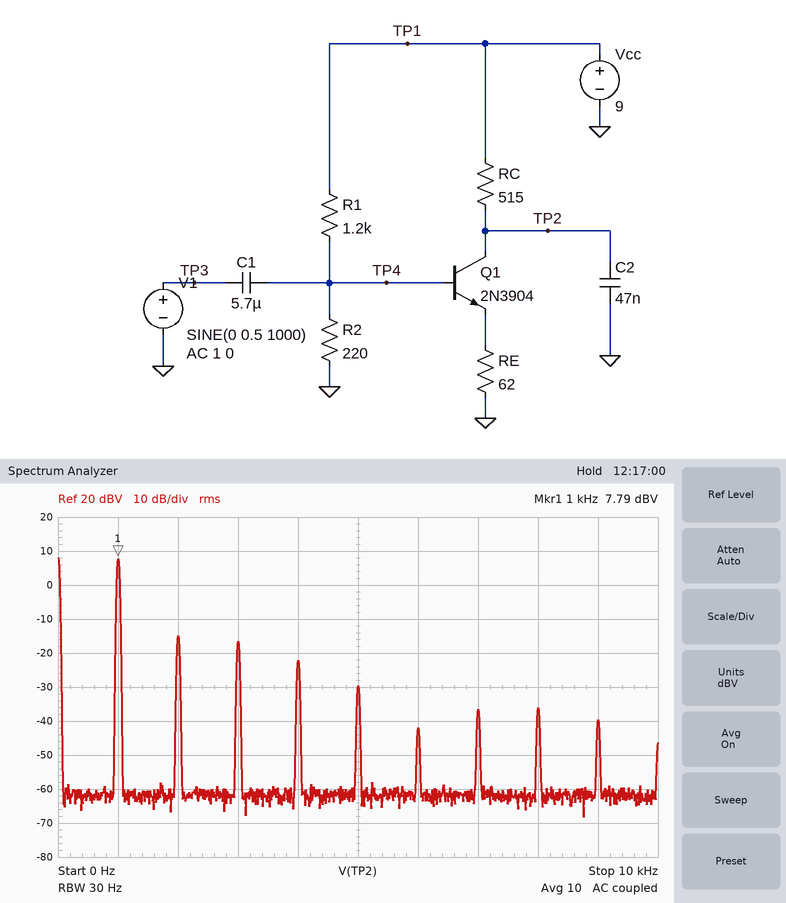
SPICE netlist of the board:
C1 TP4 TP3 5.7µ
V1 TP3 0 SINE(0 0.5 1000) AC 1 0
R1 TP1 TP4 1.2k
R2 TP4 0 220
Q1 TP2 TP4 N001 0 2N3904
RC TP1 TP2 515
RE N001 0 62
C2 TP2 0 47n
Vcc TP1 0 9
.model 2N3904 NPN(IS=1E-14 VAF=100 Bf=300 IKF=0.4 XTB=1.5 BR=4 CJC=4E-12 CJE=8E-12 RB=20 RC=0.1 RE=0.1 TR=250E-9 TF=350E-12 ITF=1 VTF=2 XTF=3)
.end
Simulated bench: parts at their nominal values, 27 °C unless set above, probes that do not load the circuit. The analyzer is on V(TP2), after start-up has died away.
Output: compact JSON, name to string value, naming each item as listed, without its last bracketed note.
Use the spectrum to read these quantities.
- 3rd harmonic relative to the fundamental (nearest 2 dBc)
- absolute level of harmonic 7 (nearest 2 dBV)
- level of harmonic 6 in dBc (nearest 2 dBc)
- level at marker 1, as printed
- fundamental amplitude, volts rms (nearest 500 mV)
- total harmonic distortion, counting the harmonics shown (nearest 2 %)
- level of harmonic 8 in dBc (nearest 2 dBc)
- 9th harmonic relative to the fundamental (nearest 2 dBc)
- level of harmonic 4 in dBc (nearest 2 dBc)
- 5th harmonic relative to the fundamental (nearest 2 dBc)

{"3rd harmonic relative to the fundamental": "-24 dBc", "absolute level of harmonic 7": "-36 dBV", "level of harmonic 6 in dBc": "-50 dBc", "level at marker 1, as printed": "7.79 dBV", "fundamental amplitude, volts rms": "2.5 V", "total harmonic distortion, counting the harmonics shown": "10 %", "level of harmonic 8 in dBc": "-44 dBc", "9th harmonic relative to the fundamental": "-48 dBc", "level of harmonic 4 in dBc": "-30 dBc", "5th harmonic relative to the fundamental": "-38 dBc"}
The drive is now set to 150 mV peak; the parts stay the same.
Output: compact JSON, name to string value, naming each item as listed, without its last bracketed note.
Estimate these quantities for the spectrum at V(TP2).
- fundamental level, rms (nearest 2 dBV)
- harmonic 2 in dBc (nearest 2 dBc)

{"fundamental level, rms": "-2 dBV", "harmonic 2 in dBc": "-54 dBc"}
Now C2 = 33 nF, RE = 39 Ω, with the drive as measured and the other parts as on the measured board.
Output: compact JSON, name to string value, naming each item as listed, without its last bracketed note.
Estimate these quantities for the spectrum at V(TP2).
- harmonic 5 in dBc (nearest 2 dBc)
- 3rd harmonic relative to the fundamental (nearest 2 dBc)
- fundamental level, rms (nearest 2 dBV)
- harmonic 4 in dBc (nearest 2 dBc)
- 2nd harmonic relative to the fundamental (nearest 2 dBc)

{"harmonic 5 in dBc": "-30 dBc", "3rd harmonic relative to the fundamental": "-20 dBc", "fundamental level, rms": "10 dBV", "harmonic 4 in dBc": "-36 dBc", "2nd harmonic relative to the fundamental": "-14 dBc"}
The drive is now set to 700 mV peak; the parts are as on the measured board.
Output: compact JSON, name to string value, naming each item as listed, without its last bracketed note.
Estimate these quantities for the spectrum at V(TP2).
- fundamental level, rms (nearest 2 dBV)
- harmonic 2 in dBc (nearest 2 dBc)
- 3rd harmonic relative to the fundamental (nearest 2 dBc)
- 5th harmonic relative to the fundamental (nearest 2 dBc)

{"fundamental level, rms": "10 dBV", "harmonic 2 in dBc": "-20 dBc", "3rd harmonic relative to the fundamental": "-20 dBc", "5th harmonic relative to the fundamental": "-42 dBc"}
